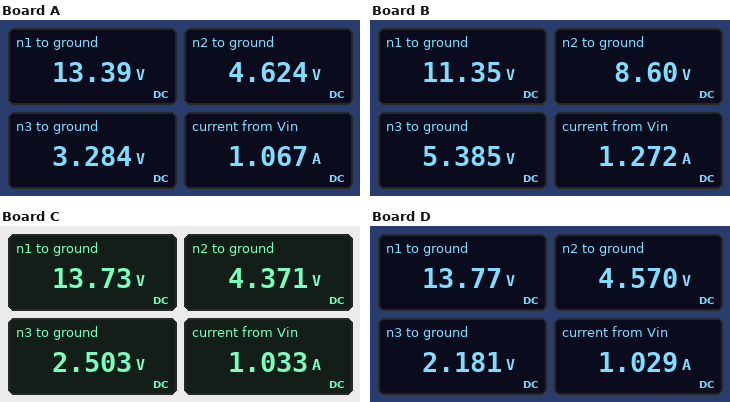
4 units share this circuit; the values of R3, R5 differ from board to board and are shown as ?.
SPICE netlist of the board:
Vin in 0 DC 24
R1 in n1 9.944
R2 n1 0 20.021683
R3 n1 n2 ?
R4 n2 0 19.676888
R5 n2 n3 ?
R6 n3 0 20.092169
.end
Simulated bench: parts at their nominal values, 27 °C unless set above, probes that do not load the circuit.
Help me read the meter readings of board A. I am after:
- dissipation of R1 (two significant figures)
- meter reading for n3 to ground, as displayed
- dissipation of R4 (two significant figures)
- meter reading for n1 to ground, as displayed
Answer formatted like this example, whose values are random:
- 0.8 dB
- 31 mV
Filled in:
- 11 W
- 3.284 V
- 1.1 W
- 13.39 V
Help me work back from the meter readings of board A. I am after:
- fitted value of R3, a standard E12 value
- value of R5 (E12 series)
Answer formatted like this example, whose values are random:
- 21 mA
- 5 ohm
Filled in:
- 22 Ω
- 8.2 Ω
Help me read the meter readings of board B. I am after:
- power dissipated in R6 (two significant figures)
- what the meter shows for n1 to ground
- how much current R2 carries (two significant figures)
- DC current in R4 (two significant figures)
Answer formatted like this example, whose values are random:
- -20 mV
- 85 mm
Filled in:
- 1.4 W
- 11.35 V
- 570 mA
- 440 mA
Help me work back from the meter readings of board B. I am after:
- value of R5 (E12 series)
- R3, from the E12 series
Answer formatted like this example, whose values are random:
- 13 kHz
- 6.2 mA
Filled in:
- 12 Ω
- 3.9 Ω
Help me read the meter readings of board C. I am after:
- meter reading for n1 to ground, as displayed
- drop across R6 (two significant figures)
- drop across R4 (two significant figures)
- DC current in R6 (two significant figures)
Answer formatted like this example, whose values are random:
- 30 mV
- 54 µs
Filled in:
- 13.73 V
- 2.5 V
- 4.4 V
- 120 mA
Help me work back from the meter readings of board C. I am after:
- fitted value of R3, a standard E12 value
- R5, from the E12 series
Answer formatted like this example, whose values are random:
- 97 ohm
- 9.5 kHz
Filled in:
- 27 Ω
- 15 Ω
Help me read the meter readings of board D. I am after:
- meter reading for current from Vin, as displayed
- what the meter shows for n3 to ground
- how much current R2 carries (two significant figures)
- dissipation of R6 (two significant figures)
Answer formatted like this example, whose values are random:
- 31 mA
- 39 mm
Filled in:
- 1.029 A
- 2.181 V
- 690 mA
- 240 mW
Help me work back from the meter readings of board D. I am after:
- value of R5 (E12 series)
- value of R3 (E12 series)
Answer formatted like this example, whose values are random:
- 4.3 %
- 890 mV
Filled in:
- 22 Ω
- 27 Ω
